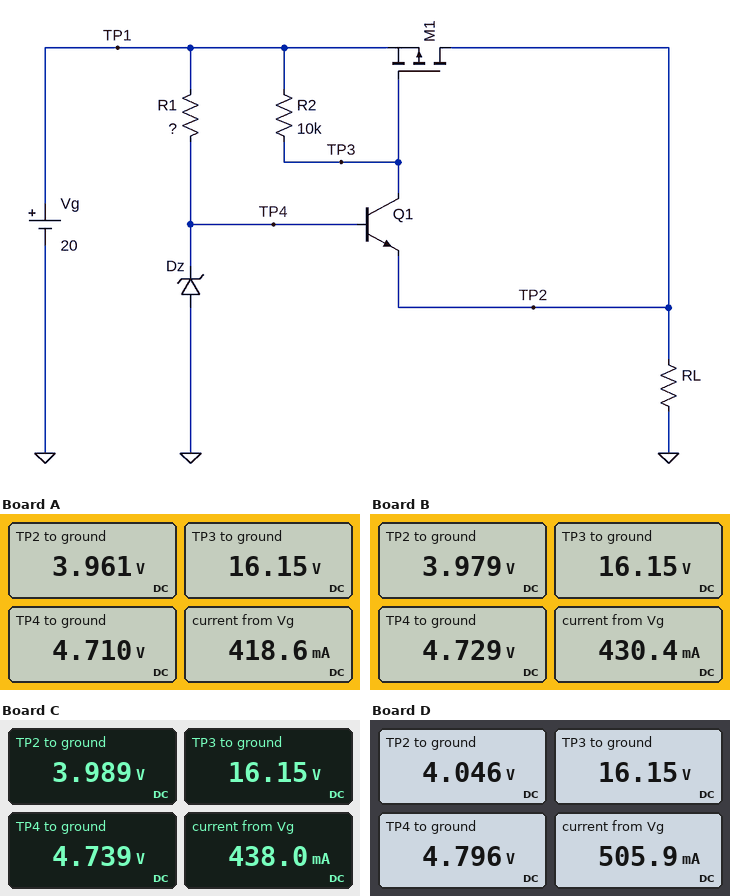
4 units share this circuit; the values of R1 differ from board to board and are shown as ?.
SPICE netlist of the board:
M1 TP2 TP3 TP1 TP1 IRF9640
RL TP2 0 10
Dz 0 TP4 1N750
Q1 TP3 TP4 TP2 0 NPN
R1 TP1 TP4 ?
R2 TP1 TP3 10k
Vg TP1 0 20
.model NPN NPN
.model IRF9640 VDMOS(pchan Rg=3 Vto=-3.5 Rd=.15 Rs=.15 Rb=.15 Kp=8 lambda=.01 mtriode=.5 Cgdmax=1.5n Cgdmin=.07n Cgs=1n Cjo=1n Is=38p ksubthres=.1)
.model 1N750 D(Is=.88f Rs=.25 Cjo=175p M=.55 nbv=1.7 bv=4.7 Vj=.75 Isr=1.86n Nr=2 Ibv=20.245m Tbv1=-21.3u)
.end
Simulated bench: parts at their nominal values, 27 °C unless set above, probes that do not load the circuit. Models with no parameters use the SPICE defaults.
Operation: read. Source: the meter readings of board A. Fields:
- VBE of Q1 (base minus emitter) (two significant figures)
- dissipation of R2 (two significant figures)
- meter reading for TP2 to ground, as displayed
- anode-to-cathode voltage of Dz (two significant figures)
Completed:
750 mV
1.5 mW
3.961 V
-4.7 V
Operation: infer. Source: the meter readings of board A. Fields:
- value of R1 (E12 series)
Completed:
680 Ω
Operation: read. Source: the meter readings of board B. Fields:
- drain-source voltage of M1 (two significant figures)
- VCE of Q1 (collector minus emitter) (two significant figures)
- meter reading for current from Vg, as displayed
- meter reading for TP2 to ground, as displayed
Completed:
-16 V
12 V
430.4 mA
3.979 V
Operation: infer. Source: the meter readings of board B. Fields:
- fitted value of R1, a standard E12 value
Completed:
470 Ω
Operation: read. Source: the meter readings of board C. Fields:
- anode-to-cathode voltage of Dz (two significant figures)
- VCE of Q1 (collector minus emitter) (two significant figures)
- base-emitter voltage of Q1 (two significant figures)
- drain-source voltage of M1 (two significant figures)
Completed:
-4.7 V
12 V
750 mV
-16 V
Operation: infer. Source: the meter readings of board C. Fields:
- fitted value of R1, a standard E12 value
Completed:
390 Ω
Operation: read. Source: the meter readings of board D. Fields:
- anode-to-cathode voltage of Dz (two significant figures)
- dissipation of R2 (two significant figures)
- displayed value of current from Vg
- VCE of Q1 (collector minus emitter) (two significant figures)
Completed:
-4.8 V
1.5 mW
505.9 mA
12 V
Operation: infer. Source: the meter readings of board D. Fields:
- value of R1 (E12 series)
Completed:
150 Ω
